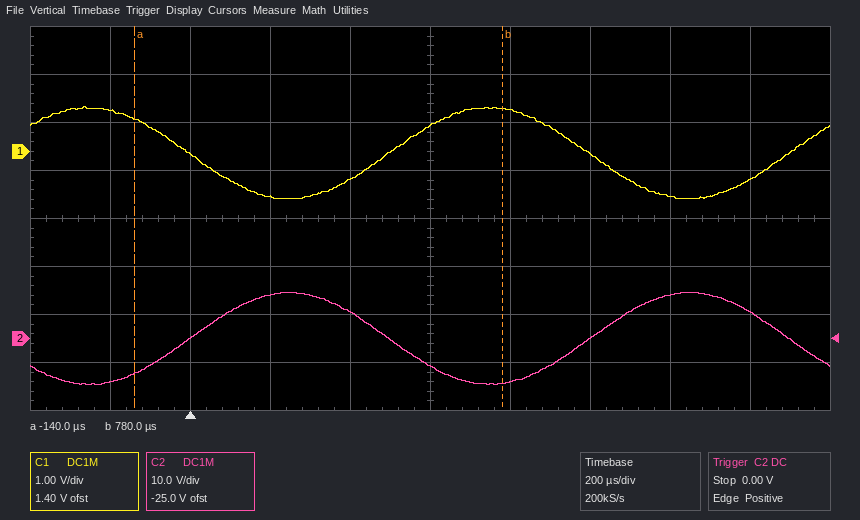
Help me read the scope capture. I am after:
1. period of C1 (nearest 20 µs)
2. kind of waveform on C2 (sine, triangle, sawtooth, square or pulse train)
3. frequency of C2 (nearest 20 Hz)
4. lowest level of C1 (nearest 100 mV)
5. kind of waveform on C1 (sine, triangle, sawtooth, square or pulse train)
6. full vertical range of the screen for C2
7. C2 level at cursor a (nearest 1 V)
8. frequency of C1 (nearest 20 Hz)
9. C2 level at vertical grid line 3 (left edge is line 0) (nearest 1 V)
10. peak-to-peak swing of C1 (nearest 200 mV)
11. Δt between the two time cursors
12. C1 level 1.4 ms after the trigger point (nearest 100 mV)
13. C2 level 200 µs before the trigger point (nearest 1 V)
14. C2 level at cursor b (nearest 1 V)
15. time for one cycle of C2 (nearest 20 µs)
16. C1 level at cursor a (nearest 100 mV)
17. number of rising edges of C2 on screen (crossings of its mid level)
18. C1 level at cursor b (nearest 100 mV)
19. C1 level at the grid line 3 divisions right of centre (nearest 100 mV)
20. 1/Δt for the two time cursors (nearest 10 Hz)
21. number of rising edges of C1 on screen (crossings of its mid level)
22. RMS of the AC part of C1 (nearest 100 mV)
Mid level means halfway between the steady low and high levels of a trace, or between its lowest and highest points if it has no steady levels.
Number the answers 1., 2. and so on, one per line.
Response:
1. 1.00 ms
2. sine
3. 1.00 kHz
4. -1.0 V
5. sine
6. 80 V
7. -7 V
8. 1.00 kHz
9. 9 V
10. 2.0 V
11. 920 µs
12. -600 mV
13. -9 V
14. -9 V
15. 1.00 ms
16. 700 mV
17. 2
18. 900 mV
19. -900 mV
20. 1.09 kHz
21. 2
22. 700 mV
